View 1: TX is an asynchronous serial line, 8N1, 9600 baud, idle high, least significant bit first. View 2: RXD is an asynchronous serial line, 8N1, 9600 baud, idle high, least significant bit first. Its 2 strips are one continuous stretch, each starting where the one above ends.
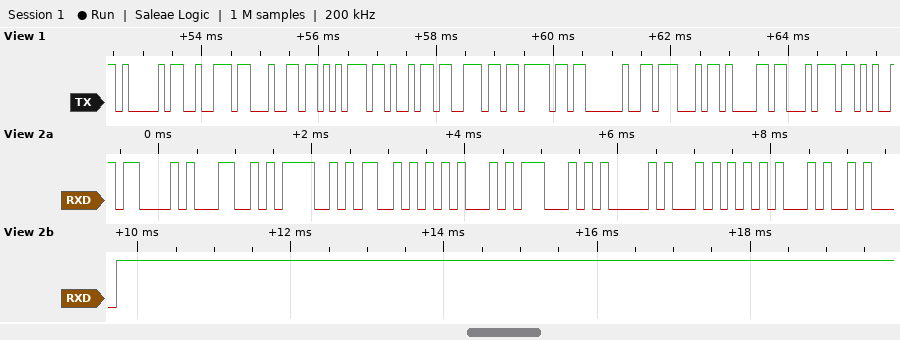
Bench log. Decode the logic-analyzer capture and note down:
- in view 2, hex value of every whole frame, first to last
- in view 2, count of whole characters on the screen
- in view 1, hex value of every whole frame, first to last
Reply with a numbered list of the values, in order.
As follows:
1. 43 4C 4F 53 45 47 41 54 45 0A
2. 10
3. 0x41 0x72 0x64 0x75 0x69 0x6E 0x6F 0x20 0x47 0x61 0x74
